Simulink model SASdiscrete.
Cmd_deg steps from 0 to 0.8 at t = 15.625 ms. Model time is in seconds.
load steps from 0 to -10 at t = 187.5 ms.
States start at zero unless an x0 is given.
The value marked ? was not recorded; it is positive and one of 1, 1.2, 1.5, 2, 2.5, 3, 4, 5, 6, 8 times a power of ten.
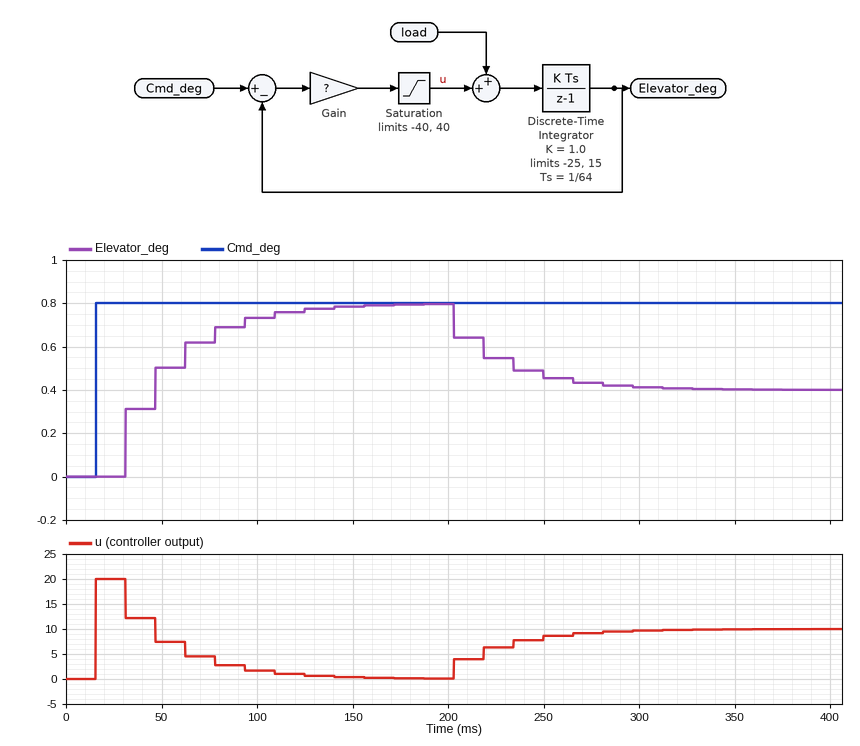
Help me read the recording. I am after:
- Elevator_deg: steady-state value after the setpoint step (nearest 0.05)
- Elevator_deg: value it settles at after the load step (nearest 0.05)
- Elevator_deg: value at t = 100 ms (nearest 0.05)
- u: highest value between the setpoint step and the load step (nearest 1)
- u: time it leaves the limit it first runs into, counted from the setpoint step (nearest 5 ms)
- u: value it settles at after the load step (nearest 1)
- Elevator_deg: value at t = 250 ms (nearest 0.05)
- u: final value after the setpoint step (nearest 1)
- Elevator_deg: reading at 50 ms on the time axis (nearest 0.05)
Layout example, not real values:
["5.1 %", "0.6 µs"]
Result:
["0.80", "0.40", "0.75", "20", "15 ms", "10", "0.45", "0", "0.50"]
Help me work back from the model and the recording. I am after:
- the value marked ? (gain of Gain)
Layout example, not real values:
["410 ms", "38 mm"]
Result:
["25"]
